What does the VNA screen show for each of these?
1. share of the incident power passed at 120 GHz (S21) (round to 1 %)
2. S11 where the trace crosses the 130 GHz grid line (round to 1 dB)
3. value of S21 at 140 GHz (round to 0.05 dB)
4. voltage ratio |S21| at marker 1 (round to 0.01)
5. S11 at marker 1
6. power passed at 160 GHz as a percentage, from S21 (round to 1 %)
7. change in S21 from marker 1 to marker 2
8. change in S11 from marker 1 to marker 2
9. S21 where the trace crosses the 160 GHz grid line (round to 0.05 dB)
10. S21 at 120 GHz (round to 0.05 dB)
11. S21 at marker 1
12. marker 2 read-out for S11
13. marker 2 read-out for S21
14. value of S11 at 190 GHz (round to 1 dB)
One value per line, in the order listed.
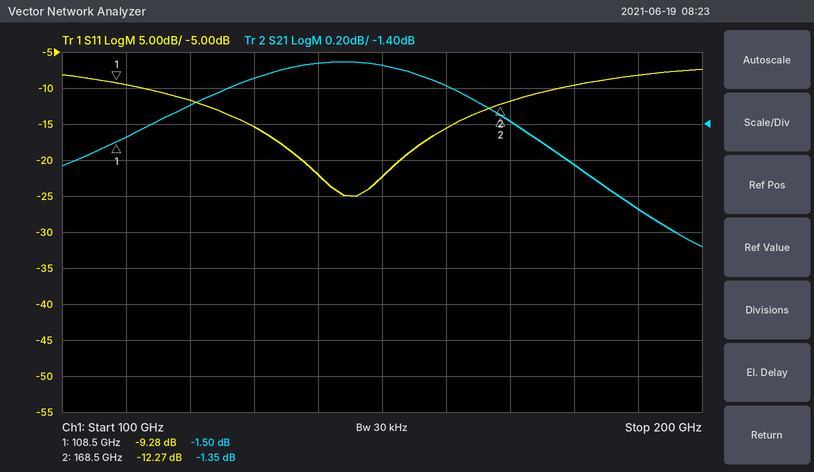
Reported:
74 %
-15 dB
-1.05 dB
0.84
-9.28 dB
76 %
0.15 dB
-2.99 dB
-1.20 dB
-1.30 dB
-1.50 dB
-12.27 dB
-1.35 dB
-8 dB
